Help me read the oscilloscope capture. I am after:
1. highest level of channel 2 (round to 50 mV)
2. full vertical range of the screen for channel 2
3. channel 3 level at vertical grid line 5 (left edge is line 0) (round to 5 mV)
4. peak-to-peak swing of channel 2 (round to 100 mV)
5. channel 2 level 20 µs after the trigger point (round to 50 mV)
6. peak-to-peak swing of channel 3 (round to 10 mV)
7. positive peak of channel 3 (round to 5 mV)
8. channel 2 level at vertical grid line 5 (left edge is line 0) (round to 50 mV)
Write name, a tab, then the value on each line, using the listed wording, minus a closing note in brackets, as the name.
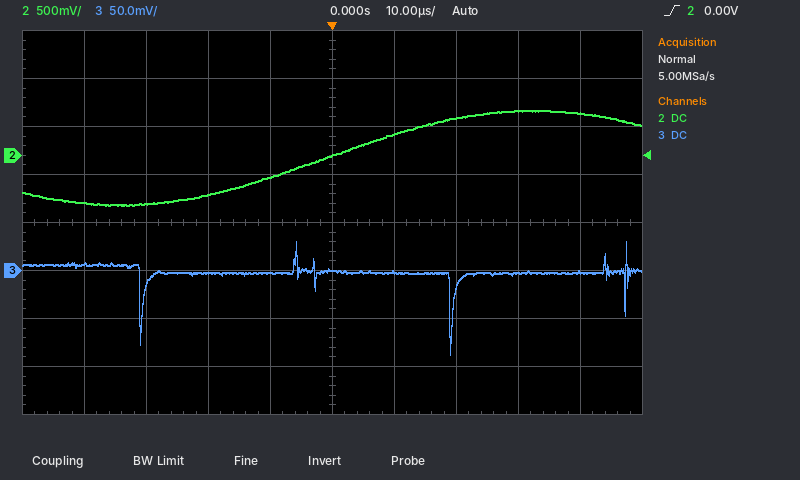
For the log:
highest level of channel 2	450 mV
full vertical range of the screen for channel 2	4 V
channel 3 level at vertical grid line 5 (left edge is line 0)	0 mV
peak-to-peak swing of channel 2	1.00 V
channel 2 level 20 µs after the trigger point	400 mV
peak-to-peak swing of channel 3	120 mV
positive peak of channel 3	30 mV
channel 2 level at vertical grid line 5 (left edge is line 0)	0 mV
